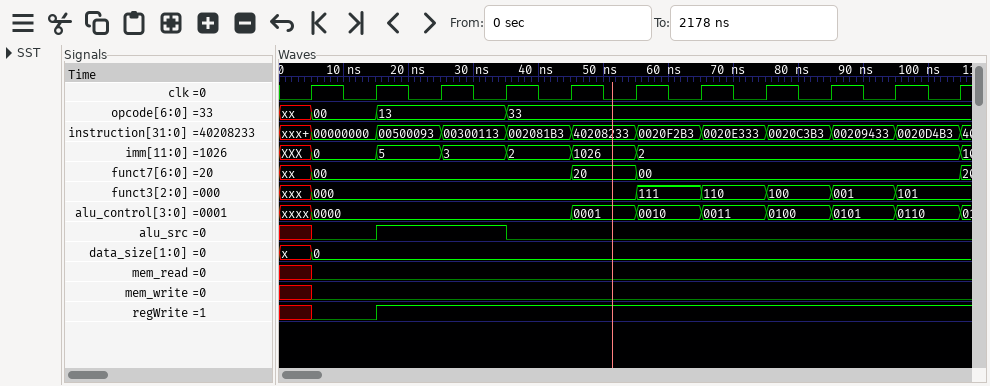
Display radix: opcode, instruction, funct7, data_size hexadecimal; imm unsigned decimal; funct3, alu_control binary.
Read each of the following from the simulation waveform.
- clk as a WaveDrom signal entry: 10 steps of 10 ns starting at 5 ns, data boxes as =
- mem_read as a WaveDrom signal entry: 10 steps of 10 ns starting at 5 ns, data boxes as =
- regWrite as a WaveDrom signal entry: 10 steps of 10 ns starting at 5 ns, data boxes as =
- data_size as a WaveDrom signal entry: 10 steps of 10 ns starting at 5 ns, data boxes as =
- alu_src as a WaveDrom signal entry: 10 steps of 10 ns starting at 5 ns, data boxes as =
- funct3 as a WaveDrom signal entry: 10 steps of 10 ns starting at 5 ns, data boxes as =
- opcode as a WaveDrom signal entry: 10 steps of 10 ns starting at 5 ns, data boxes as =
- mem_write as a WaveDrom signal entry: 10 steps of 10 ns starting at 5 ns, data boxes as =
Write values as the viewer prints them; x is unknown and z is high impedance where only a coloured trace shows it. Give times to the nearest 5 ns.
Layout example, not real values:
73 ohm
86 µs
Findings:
{name: 'clk', wave: 'p.........'}
{name: 'mem_read', wave: '0.........'}
{name: 'regWrite', wave: '01........'}
{name: 'data_size', wave: '=.........', data: '0'}
{name: 'alu_src', wave: '01.0......'}
{name: 'funct3', wave: '=....=====', data: '000 111 110 100 001 101'}
{name: 'opcode', wave: '==.=......', data: '00 13 33'}
{name: 'mem_write', wave: '0.........'}
